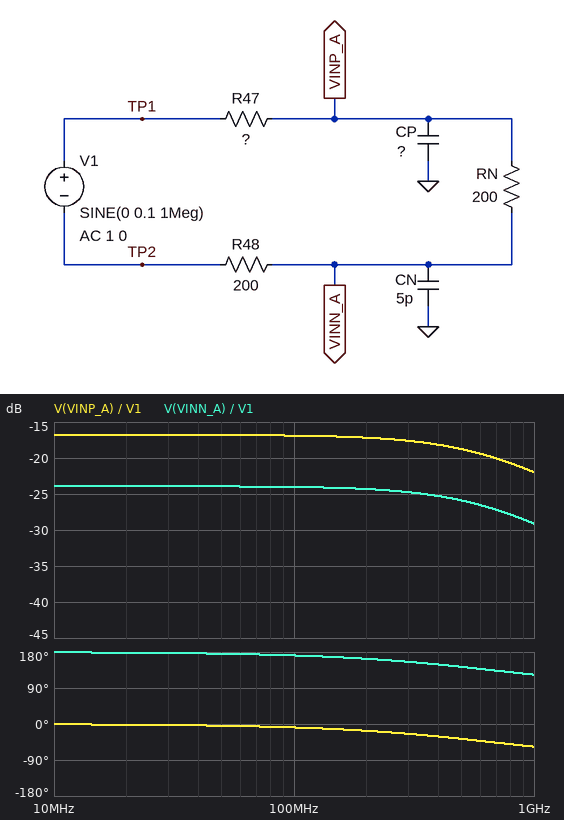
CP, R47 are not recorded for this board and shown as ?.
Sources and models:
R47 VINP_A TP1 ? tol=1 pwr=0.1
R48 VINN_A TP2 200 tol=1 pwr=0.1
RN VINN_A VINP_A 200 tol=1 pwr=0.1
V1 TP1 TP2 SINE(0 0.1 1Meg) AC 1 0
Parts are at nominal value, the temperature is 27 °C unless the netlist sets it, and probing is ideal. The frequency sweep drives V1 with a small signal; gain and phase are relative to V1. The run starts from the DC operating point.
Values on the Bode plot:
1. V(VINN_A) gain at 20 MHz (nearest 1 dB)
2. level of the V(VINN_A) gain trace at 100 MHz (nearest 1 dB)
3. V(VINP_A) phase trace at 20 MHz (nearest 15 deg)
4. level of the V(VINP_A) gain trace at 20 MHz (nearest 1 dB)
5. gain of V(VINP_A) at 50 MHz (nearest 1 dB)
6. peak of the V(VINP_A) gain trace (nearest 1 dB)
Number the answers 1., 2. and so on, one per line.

1. -24 dB
2. -24 dB
3. 0 deg
4. -17 dB
5. -17 dB
6. -17 dB
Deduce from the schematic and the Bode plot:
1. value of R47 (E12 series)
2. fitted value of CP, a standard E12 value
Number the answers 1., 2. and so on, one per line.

1. 560 Ω
2. 2.2 pF
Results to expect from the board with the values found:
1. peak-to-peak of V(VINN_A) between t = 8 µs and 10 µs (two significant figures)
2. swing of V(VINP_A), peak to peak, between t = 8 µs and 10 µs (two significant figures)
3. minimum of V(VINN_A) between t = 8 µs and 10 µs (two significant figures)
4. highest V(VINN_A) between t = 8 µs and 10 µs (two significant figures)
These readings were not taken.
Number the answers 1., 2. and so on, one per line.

1. 13 mV
2. 29 mV
3. -6.4 mV
4. 6.4 mV
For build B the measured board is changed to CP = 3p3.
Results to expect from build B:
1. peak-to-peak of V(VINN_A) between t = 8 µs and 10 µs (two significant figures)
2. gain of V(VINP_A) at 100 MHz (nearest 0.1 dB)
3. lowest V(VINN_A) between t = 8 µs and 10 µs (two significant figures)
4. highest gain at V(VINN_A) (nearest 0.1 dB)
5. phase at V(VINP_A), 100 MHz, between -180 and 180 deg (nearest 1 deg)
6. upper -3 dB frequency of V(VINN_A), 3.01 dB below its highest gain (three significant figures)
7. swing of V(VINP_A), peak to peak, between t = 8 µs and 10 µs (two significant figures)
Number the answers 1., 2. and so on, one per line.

1. 17 mV
2. -18.2 dB
3. -8.3 mV
4. -21.6 dB
5. -11 deg
6. 506 MHz
7. 25 mV
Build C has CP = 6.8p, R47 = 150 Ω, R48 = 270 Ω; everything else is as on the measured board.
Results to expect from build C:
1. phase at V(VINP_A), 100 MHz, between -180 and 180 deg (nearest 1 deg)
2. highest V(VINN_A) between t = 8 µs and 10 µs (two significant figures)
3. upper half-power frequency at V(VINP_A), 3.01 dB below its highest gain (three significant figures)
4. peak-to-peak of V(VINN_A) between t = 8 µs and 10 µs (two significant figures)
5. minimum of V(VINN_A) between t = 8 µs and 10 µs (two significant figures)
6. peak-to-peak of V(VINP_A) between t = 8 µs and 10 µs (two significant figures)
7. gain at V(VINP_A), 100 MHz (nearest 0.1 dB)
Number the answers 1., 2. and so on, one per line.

1. -14 deg
2. 19 mV
3. 408 MHz
4. 37 mV
5. -19 mV
6. 27 mV
7. -17.5 dB
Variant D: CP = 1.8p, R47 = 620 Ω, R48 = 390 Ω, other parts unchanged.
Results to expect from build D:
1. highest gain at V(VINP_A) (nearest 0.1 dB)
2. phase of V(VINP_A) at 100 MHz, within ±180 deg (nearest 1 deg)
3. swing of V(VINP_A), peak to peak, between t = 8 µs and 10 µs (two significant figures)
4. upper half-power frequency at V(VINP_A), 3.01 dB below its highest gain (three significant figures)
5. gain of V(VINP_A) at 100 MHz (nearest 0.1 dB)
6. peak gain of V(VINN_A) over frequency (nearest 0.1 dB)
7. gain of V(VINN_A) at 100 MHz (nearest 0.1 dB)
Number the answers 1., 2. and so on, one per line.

1. -18.3 dB
2. -8 deg
3. 24 mV
4. 720 MHz
5. -18.4 dB
6. -27.2 dB
7. -27.3 dB
